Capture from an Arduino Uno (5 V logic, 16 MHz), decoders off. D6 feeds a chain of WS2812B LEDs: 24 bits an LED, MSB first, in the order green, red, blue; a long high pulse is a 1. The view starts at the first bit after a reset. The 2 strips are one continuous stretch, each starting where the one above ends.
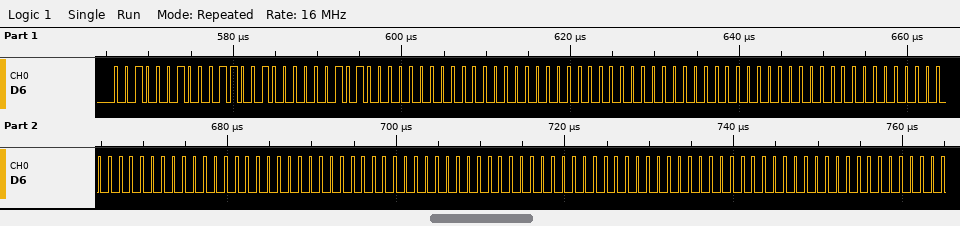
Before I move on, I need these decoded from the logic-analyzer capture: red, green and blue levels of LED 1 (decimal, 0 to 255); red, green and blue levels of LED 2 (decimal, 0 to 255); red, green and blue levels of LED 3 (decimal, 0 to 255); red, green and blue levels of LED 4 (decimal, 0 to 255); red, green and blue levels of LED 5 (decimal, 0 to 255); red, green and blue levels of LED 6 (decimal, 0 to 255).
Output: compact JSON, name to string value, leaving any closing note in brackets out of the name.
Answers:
{"red, green and blue levels of LED 1": "50, 34, 5", "red, green and blue levels of LED 2": "0, 0, 0", "red, green and blue levels of LED 3": "0, 0, 0", "red, green and blue levels of LED 4": "0, 0, 0", "red, green and blue levels of LED 5": "0, 0, 0", "red, green and blue levels of LED 6": "0, 0, 0"}
